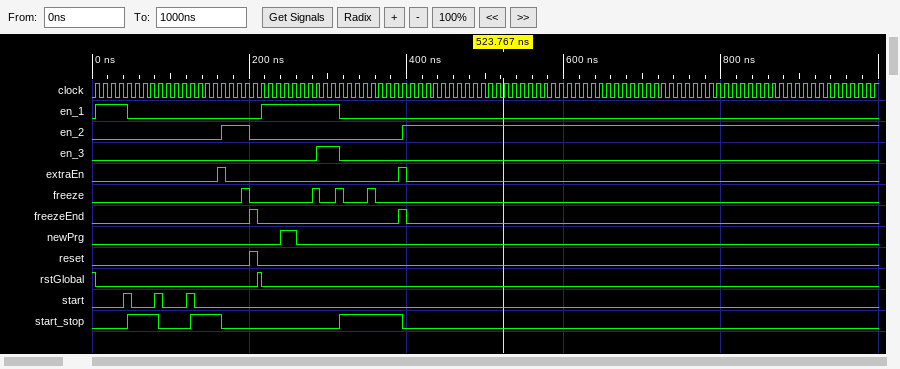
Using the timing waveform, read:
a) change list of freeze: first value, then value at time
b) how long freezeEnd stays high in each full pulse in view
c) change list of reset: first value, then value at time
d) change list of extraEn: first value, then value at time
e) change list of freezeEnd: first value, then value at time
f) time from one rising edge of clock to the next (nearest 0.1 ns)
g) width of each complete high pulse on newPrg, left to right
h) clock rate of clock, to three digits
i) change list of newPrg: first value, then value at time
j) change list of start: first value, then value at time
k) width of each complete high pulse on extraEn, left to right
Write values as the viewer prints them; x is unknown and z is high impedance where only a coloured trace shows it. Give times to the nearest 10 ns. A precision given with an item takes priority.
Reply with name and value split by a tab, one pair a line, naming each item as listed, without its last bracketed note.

change list of freeze: first value, then value at time	0, 1 at 190 ns, 0 at 200 ns, 1 at 280 ns, 0 at 290 ns, 1 at 310 ns, 0 at 320 ns, 1 at 350 ns, 0 at 360 ns
how long freezeEnd stays high in each full pulse in view	10 ns, 10 ns
change list of reset: first value, then value at time	0, 1 at 200 ns, 0 at 210 ns
change list of extraEn: first value, then value at time	0, 1 at 160 ns, 0 at 170 ns, 1 at 390 ns, 0 at 400 ns
change list of freezeEnd: first value, then value at time	0, 1 at 200 ns, 0 at 210 ns, 1 at 390 ns, 0 at 400 ns
time from one rising edge of clock to the next	10 ns
width of each complete high pulse on newPrg, left to right	20 ns
clock rate of clock, to three digits	100 MHz
change list of newPrg: first value, then value at time	0, 1 at 240 ns, 0 at 260 ns
change list of start: first value, then value at time	0, 1 at 40 ns, 0 at 50 ns, 1 at 80 ns, 0 at 90 ns, 1 at 120 ns, 0 at 130 ns
width of each complete high pulse on extraEn, left to right	10 ns, 10 ns
